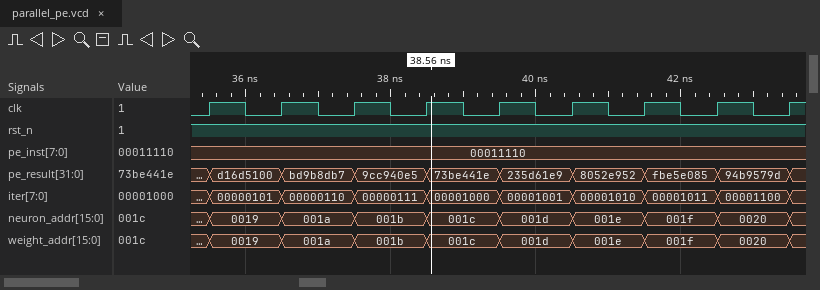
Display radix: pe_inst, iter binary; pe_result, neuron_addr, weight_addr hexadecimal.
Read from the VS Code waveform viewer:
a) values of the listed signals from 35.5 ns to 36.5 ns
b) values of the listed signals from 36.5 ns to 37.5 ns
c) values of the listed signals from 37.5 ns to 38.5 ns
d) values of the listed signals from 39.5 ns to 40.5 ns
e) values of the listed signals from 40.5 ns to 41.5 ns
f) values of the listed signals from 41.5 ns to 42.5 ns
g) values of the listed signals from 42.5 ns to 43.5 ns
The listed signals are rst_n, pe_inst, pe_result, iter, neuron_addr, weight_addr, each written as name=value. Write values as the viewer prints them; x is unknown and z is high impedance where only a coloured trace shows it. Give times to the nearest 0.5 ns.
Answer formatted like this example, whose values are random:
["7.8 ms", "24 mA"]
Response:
["rst_n=1, pe_inst=00011110, pe_result=d16d5100, iter=00000101, neuron_addr=0019, weight_addr=0019", "rst_n=1, pe_inst=00011110, pe_result=bd9b8db7, iter=00000110, neuron_addr=001a, weight_addr=001a", "rst_n=1, pe_inst=00011110, pe_result=9cc940e5, iter=00000111, neuron_addr=001b, weight_addr=001b", "rst_n=1, pe_inst=00011110, pe_result=235d61e9, iter=00001001, neuron_addr=001d, weight_addr=001d", "rst_n=1, pe_inst=00011110, pe_result=8052e952, iter=00001010, neuron_addr=001e, weight_addr=001e", "rst_n=1, pe_inst=00011110, pe_result=fbe5e085, iter=00001011, neuron_addr=001f, weight_addr=001f", "rst_n=1, pe_inst=00011110, pe_result=94b9579d, iter=00001100, neuron_addr=0020, weight_addr=0020"]
